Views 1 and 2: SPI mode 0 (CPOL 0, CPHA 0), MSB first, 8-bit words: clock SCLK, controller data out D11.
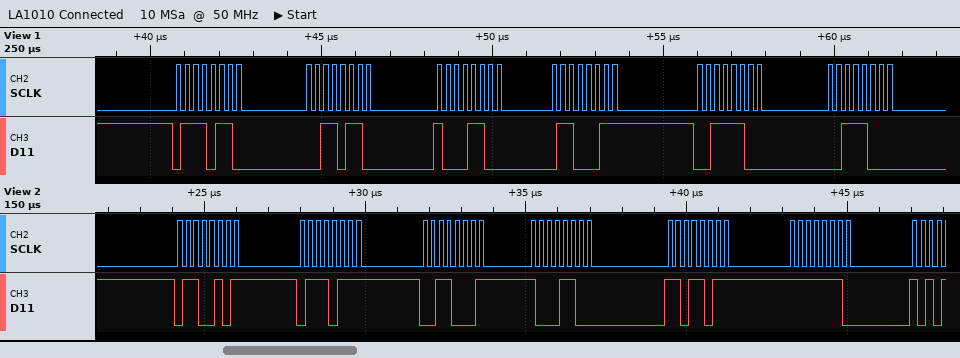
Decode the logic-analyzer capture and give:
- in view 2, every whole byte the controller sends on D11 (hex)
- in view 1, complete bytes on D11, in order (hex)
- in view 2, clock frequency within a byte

0x65 0x77 0x31 0x8C 0xDB 0xFE
76 36 8C 63 3C 38
4 MHz
